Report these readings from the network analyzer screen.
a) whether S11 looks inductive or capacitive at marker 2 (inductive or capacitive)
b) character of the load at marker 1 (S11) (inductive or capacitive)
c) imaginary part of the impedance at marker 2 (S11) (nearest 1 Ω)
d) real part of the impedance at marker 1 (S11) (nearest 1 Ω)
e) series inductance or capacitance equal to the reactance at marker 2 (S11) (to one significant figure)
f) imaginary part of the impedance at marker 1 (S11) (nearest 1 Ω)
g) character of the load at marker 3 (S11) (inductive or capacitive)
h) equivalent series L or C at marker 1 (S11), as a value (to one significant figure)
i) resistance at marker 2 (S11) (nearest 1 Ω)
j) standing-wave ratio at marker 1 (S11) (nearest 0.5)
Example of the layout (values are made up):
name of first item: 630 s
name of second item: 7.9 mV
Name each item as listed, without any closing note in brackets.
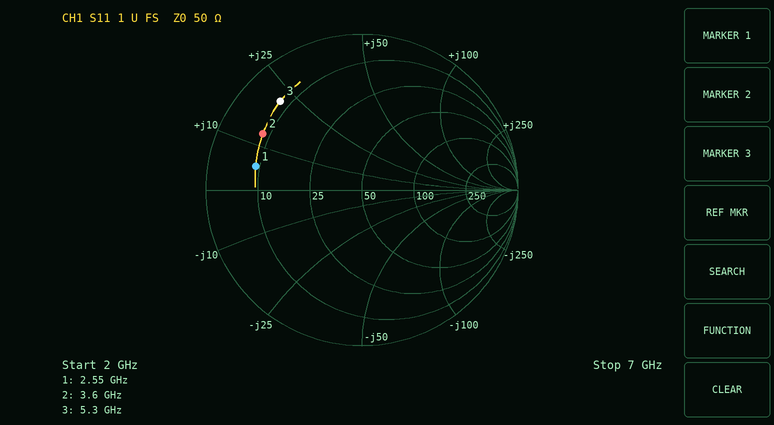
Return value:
whether S11 looks inductive or capacitive at marker 2: inductive
character of the load at marker 1 (S11): inductive
imaginary part of the impedance at marker 2 (S11): +13 Ω
real part of the impedance at marker 1 (S11): 9 Ω
series inductance or capacitance equal to the reactance at marker 2 (S11): 600 pH
imaginary part of the impedance at marker 1 (S11): +5 Ω
character of the load at marker 3 (S11): inductive
equivalent series L or C at marker 1 (S11), as a value: 300 pH
resistance at marker 2 (S11): 8 Ω
standing-wave ratio at marker 1 (S11): 5.5
